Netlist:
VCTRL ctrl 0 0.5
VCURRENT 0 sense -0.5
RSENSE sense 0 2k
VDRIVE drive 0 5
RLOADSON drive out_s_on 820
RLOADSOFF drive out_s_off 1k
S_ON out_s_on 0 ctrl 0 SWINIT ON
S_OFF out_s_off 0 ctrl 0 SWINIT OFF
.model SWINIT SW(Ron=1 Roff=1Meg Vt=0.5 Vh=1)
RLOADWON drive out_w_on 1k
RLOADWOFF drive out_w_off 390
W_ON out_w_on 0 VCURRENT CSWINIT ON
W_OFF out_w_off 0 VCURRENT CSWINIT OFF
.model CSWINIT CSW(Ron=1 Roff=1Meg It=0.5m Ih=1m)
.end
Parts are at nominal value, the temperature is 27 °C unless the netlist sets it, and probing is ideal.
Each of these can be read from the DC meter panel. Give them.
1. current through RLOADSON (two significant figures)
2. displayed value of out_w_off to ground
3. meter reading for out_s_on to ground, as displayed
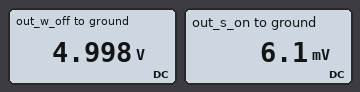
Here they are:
6.1 mA
4.998 V
6.1 mV
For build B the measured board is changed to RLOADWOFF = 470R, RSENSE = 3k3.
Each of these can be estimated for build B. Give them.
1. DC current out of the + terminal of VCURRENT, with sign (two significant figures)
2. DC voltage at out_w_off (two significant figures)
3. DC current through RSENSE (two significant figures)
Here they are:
-150 µA
5.0 V
150 µA
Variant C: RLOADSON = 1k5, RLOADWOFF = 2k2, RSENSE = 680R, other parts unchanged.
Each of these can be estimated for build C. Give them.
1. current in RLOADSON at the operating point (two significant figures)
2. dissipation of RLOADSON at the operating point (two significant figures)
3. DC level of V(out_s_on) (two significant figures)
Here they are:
3.3 mA
17 mW
3.3 mV
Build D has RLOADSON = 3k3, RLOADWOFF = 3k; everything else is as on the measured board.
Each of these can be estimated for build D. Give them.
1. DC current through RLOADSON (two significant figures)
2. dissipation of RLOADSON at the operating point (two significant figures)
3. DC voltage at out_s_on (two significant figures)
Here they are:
1.5 mA
7.6 mW
1.5 mV
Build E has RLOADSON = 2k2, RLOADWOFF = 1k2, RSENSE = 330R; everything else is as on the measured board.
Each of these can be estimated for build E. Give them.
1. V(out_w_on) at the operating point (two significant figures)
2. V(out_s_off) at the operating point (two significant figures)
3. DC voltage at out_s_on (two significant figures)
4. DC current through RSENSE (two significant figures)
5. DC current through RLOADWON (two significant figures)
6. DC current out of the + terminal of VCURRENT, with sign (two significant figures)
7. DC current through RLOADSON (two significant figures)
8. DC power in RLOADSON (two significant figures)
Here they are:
5.0 mV
5.0 V
2.3 mV
1.5 mA
5.0 mA
-1.5 mA
2.3 mA
11 mW
